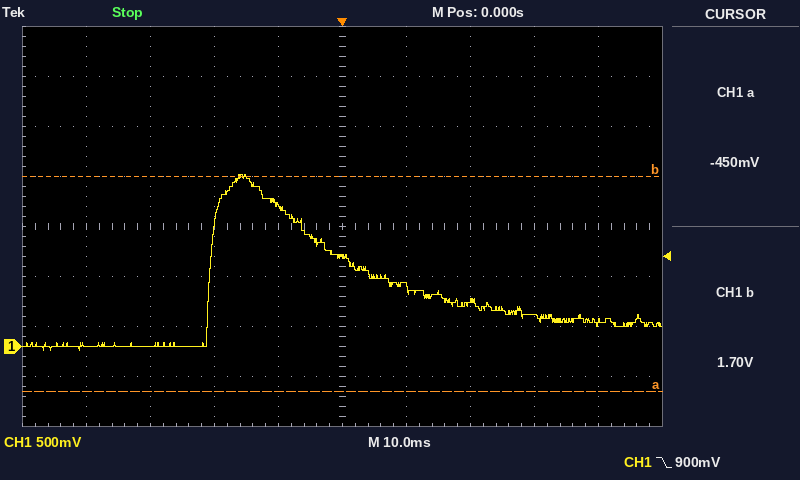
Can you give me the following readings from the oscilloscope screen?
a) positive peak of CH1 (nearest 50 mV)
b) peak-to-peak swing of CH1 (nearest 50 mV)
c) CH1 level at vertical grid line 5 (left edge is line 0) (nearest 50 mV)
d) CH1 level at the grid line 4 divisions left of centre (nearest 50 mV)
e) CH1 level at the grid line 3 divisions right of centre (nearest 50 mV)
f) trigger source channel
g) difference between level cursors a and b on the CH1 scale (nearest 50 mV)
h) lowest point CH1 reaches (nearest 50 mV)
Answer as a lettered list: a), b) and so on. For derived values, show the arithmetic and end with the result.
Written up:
a) 1.70 V
b) 1.70 V − (-50 mV) = 1.75 V
c) 900 mV
d) 0 mV
e) 300 mV
f) CH1
g) 2.15 V
h) -50 mV
